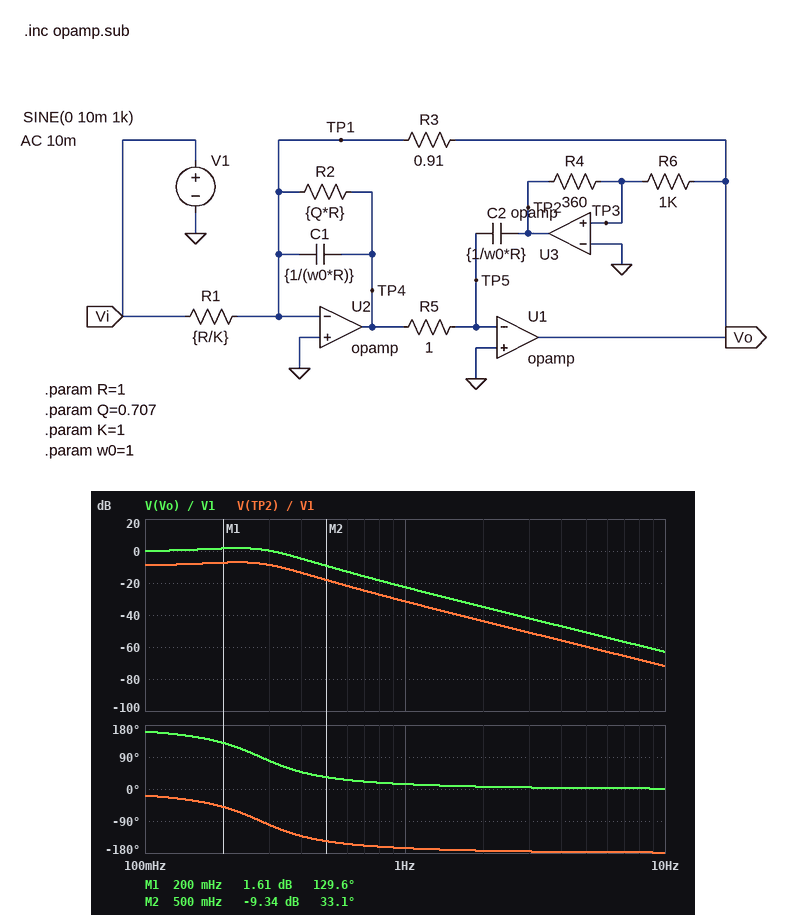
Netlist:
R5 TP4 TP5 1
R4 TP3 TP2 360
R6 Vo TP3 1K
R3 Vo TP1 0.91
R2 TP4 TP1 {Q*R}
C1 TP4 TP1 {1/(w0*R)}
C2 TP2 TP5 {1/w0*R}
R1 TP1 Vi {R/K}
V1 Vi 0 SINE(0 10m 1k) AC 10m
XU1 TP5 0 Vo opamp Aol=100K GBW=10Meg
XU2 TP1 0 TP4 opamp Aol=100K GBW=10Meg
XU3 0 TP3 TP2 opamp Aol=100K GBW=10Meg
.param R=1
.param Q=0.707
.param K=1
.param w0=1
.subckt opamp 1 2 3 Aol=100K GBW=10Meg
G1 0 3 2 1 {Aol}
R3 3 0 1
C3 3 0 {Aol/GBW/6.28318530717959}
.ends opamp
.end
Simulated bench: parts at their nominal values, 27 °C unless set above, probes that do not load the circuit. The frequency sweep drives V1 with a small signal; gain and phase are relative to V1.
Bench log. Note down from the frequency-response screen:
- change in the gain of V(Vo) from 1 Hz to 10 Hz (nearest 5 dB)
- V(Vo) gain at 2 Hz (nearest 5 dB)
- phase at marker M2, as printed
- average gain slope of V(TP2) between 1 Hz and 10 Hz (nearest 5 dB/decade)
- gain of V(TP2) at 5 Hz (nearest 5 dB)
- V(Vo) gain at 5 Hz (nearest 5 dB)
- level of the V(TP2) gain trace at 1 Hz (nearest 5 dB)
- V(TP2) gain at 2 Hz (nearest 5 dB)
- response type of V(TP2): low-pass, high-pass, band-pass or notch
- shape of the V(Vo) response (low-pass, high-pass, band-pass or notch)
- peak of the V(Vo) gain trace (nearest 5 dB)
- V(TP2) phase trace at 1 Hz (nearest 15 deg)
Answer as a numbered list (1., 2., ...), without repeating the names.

1. -40 dB
2. -35 dB
3. 33.1 deg
4. -40 dB/decade
5. -60 dB
6. -50 dB
7. -30 dB
8. -45 dB
9. low-pass
10. low-pass
11. 0 dB
12. -165 deg
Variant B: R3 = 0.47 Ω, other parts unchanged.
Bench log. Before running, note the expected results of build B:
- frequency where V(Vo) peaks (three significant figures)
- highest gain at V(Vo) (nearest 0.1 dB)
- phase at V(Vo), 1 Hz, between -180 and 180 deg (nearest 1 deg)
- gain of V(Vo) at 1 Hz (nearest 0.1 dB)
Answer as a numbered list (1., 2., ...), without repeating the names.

1. 353 mHz
2. -1.5 dB
3. 15 deg
4. -21.9 dB
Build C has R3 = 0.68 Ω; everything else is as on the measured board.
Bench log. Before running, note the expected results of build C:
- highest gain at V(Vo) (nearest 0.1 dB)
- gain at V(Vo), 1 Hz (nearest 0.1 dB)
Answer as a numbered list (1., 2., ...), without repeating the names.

1. 0.3 dB
2. -22.4 dB
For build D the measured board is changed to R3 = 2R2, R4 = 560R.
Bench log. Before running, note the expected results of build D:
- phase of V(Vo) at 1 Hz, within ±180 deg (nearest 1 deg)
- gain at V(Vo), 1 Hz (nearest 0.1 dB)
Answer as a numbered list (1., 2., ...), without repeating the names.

1. 13 deg
2. -26.9 dB
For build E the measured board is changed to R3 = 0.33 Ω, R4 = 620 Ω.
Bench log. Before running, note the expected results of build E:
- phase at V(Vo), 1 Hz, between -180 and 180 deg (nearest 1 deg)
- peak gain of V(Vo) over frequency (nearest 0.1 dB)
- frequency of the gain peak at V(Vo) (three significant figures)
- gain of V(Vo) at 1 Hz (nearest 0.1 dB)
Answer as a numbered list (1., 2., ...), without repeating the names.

1. 14 deg
2. -5.3 dB
3. 314 mHz
4. -26.9 dB
